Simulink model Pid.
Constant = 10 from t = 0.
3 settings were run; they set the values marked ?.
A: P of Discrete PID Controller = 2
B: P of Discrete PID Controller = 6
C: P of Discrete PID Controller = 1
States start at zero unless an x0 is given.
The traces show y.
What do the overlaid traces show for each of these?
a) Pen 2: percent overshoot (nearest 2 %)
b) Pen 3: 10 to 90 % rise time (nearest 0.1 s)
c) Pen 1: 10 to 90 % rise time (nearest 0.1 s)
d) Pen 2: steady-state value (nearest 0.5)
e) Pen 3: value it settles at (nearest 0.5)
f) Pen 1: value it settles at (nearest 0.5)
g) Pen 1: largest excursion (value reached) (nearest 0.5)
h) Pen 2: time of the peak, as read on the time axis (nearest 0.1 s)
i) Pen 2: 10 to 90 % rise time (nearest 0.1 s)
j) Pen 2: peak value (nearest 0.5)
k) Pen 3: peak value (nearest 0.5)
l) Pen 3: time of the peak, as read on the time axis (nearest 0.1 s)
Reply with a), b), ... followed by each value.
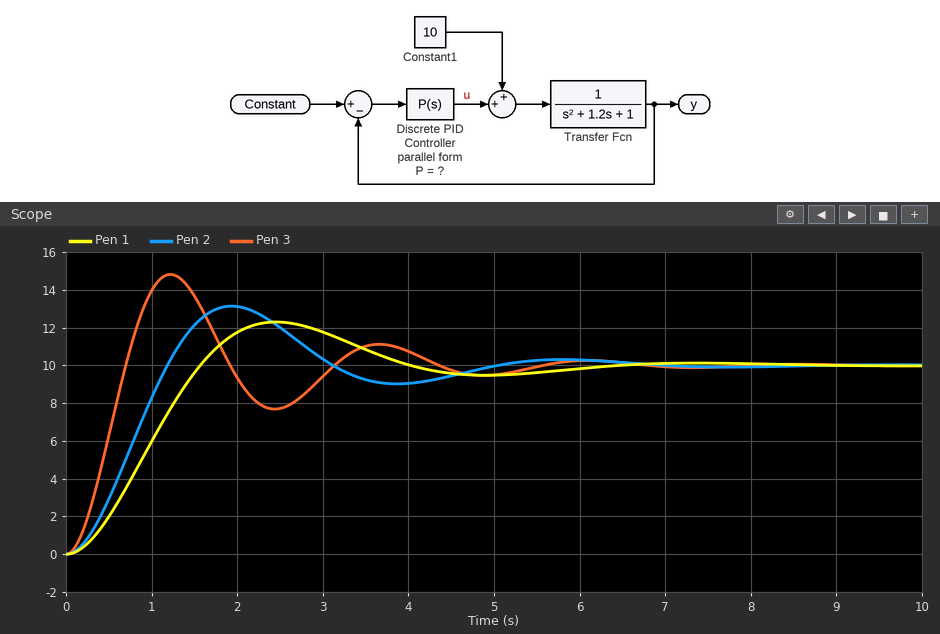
a) 32 %
b) 0.5 s
c) 1.1 s
d) 10.0
e) 10.0
f) 10.0
g) 12.5
h) 1.9 s
i) 0.8 s
j) 13.0
k) 15.0
l) 1.2 s
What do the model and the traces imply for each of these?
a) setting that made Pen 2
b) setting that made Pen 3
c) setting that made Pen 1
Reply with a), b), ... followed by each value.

a) A
b) B
c) C
